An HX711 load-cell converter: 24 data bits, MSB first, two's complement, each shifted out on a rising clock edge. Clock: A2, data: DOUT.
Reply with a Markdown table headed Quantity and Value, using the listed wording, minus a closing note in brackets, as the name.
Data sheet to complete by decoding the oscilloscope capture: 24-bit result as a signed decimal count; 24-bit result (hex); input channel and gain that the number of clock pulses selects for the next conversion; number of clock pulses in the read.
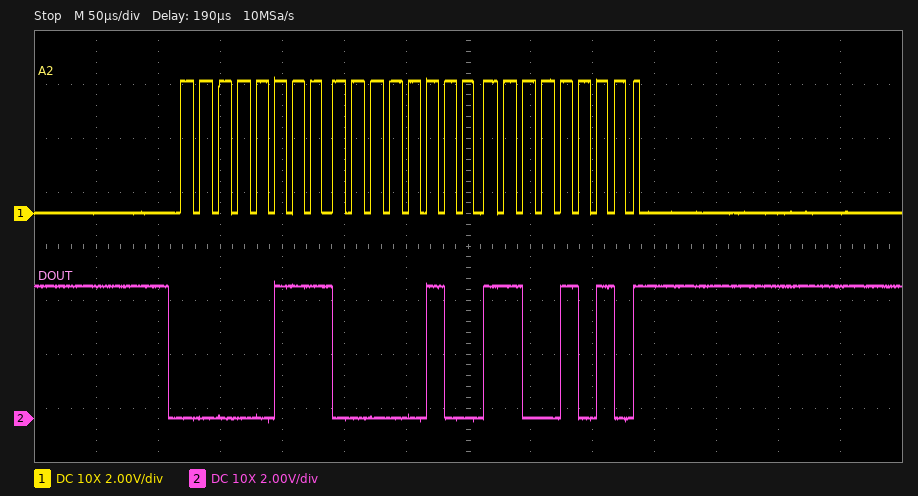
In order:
| Quantity | Value |
|---|---|
| 24-bit result as a signed decimal count | 459978 |
| 24-bit result | 0x0704CA |
| input channel and gain that the number of clock pulses selects for the next conversion | channel A, gain 128 |
| number of clock pulses in the read | 25 |
